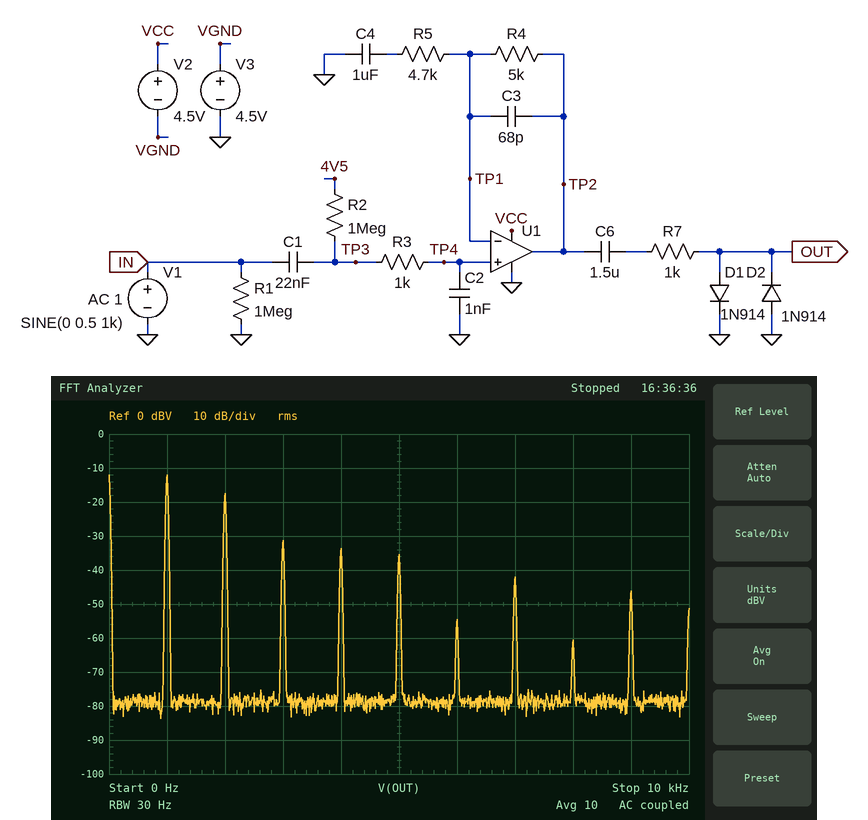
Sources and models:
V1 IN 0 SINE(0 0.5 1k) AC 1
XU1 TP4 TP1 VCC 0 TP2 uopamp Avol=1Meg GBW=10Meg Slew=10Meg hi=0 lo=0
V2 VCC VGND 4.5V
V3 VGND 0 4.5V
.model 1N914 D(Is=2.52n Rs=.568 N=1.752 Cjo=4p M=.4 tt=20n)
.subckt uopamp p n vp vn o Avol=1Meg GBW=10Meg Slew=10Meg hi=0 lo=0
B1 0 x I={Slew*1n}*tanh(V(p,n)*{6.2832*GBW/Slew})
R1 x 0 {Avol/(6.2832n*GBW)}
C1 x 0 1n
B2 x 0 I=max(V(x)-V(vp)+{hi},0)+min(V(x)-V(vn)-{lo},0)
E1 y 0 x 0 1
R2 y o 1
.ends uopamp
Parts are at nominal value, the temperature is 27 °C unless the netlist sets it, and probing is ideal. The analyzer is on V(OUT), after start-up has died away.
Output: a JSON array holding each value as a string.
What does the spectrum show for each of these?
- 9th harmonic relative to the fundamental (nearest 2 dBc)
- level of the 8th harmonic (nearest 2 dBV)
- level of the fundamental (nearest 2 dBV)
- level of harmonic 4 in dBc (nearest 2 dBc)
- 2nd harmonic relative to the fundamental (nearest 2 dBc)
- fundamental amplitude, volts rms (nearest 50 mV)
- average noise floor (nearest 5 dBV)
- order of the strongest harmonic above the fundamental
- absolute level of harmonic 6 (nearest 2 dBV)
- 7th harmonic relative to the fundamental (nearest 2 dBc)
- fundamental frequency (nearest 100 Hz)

["-34 dBc", "-60 dBV", "-12 dBV", "-22 dBc", "-6 dBc", "250 mV", "-80 dBV", "2", "-54 dBV", "-30 dBc", "1.0 kHz"]
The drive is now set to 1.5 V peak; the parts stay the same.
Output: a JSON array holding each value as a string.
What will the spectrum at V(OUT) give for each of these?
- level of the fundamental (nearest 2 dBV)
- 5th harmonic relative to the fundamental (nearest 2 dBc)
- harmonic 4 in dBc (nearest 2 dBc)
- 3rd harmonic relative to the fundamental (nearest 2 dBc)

["-8 dBV", "-16 dBc", "-14 dBc", "-36 dBc"]
